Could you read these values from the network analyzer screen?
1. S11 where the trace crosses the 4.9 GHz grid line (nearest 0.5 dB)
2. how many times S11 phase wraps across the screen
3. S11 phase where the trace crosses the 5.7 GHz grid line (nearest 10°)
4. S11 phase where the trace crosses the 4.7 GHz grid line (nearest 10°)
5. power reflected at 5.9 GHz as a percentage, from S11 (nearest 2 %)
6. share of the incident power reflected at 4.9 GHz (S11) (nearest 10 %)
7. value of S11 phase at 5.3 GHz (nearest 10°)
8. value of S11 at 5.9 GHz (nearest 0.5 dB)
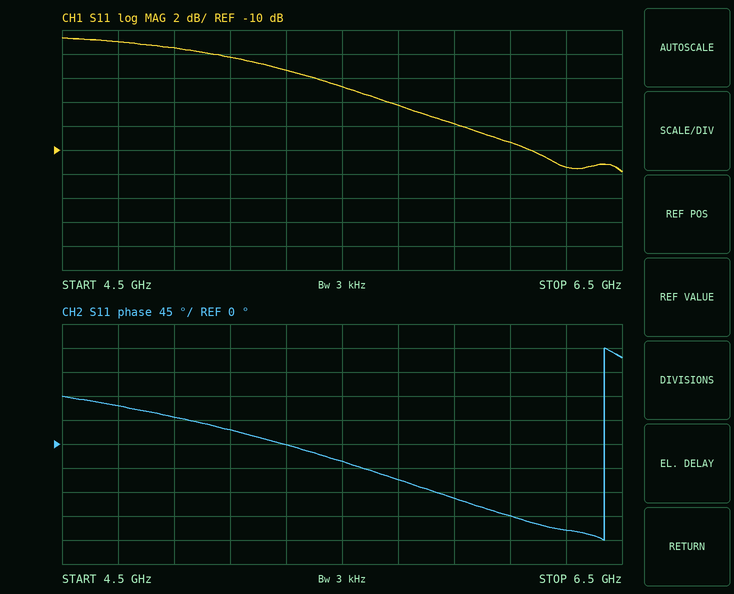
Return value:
-1.5 dB
1
-70°
70°
16 %
70 %
0°
-8.0 dB
